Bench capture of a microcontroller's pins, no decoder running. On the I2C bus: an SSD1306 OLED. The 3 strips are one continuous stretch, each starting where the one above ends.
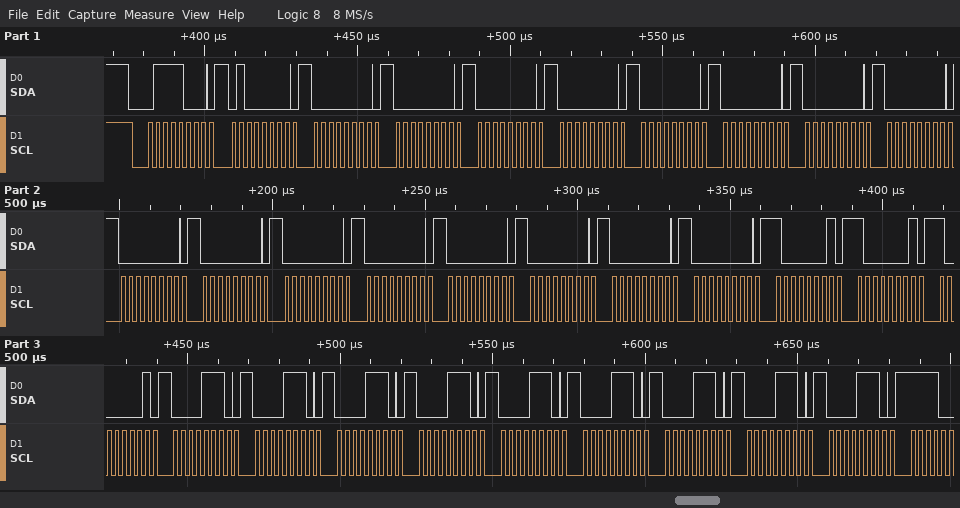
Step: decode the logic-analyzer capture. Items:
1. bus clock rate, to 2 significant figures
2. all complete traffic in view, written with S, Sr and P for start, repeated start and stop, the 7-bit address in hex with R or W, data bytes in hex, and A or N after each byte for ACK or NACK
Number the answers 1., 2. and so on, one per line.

1. 400 kHz
2. S 3CW A 40 A 00 A 00 A 00 A 00 A 00 A 00 A 00 A 00 A 00 A 00 A 00 A 00 A 00 A 00 A 00 A 00 A 81 A 81 A 81 A 0E A 0E A 0E A 0E A 0E A 0E A 0E A 0E A 0E A
